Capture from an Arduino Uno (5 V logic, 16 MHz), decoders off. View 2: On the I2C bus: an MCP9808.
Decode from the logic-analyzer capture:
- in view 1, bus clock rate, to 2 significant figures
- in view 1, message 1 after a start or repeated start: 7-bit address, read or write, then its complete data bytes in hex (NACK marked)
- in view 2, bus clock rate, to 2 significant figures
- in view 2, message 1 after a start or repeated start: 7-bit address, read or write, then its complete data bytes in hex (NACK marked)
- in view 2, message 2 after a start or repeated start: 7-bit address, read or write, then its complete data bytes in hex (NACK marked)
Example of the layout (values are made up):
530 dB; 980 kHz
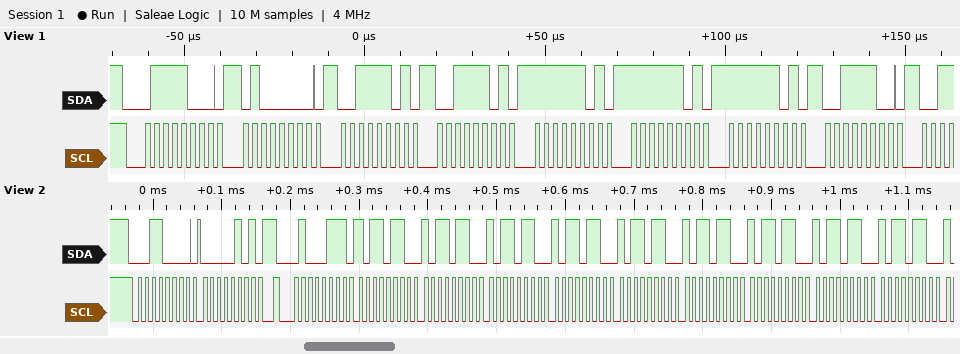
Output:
400 kHz; 0x3C write: 40 3D 3D FD FD FD 3C; 100 kHz; 0x18 write: 05; 0x23 read: B6 B6 B6 B6 B6 B6 B6 B6 B6
